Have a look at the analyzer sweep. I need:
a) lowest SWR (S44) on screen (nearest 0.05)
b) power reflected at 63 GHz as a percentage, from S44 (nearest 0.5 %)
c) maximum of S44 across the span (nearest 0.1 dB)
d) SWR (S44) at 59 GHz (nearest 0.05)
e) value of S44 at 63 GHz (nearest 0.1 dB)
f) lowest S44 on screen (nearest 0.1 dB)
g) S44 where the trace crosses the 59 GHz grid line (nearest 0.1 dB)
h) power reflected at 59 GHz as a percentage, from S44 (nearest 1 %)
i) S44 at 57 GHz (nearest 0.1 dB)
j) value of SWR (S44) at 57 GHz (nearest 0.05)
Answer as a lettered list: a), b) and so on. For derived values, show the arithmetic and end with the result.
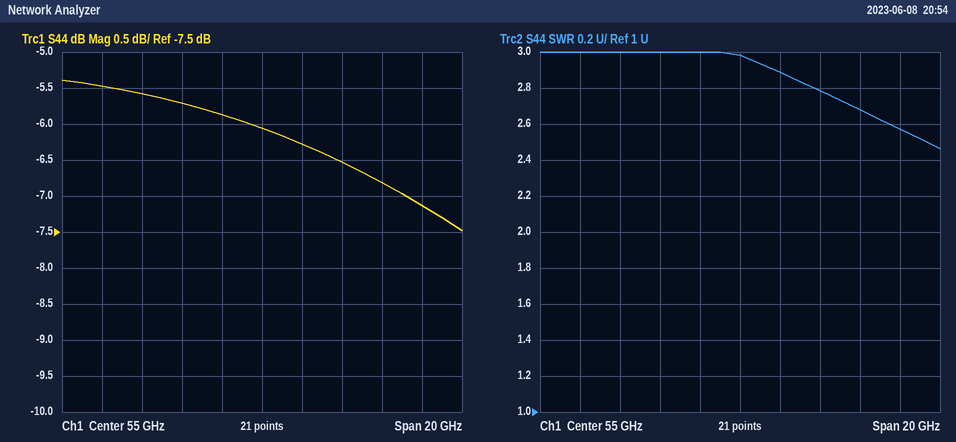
a) 2.45
b) 10^(-7.1/10) ≈ 19.5 %
c) -5.4 dB
d) 2.80
e) -7.1 dB
f) -7.5 dB
g) -6.5 dB
h) 10^(-6.5/10) ≈ 22 %
i) -6.3 dB
j) 2.90
